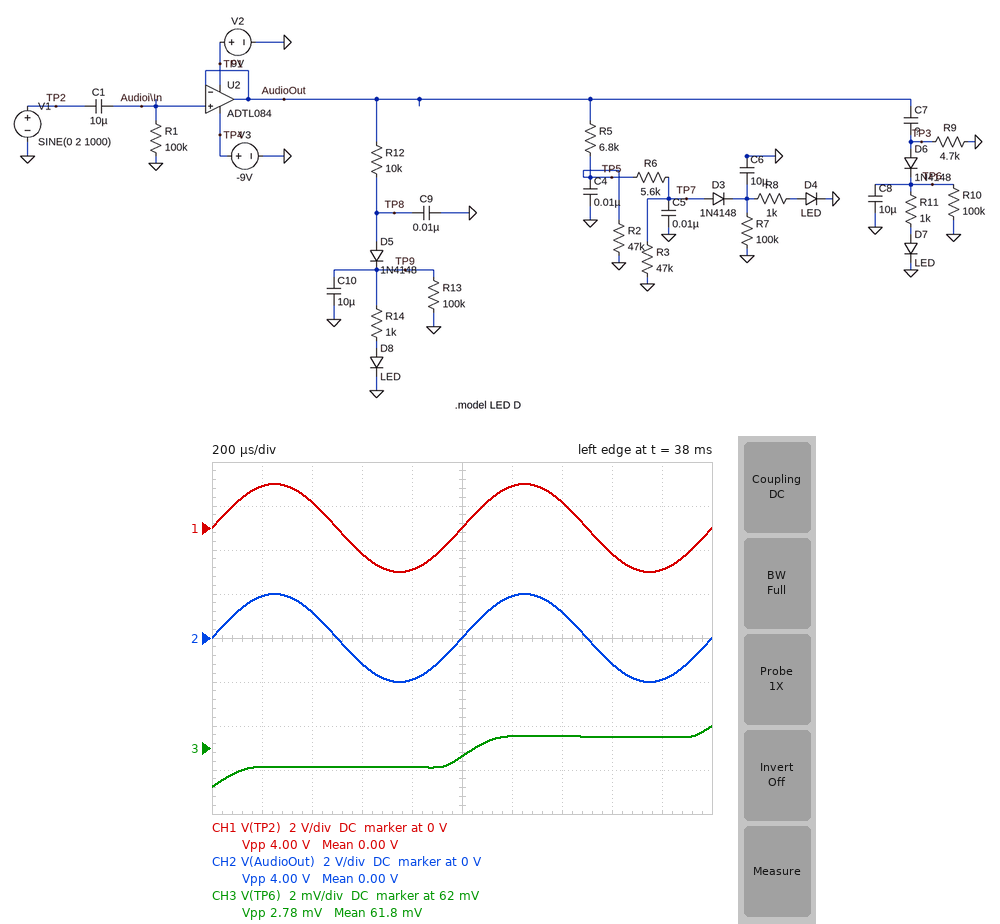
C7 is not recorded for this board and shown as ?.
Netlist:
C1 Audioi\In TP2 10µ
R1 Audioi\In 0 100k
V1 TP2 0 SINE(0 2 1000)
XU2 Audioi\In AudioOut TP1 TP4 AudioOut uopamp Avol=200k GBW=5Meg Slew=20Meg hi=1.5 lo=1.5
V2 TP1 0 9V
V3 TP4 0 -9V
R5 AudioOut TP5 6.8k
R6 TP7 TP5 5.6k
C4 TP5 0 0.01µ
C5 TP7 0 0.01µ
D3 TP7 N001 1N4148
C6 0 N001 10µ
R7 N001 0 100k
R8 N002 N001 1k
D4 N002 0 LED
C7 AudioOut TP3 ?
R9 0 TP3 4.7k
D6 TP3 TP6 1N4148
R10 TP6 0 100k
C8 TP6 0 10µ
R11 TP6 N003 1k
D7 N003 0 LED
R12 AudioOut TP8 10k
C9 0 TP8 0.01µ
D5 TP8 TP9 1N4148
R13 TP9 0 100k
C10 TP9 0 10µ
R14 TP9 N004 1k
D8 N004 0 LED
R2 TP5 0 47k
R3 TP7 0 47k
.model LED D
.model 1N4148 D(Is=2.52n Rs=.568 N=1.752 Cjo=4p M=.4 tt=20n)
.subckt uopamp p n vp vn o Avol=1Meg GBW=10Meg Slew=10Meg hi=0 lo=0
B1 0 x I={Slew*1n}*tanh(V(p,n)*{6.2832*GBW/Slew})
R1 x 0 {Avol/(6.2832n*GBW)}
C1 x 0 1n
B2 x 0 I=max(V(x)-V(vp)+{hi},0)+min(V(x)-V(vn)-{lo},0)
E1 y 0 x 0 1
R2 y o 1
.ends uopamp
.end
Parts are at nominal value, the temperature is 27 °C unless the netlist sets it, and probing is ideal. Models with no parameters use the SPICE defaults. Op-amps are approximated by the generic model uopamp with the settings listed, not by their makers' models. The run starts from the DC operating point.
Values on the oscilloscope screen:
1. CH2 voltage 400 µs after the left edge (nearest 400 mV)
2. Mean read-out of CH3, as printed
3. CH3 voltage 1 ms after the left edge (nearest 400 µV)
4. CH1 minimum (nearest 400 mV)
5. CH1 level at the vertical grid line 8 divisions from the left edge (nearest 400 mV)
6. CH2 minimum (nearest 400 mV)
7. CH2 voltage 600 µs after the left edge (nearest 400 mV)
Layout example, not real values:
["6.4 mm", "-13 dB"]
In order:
["1.2 V", "61.8 mV", "61.6 mV", "-2.0 V", "-1.2 V", "-2.0 V", "-1.2 V"]
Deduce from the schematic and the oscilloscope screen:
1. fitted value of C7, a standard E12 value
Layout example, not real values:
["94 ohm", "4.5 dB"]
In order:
["15 nF"]
